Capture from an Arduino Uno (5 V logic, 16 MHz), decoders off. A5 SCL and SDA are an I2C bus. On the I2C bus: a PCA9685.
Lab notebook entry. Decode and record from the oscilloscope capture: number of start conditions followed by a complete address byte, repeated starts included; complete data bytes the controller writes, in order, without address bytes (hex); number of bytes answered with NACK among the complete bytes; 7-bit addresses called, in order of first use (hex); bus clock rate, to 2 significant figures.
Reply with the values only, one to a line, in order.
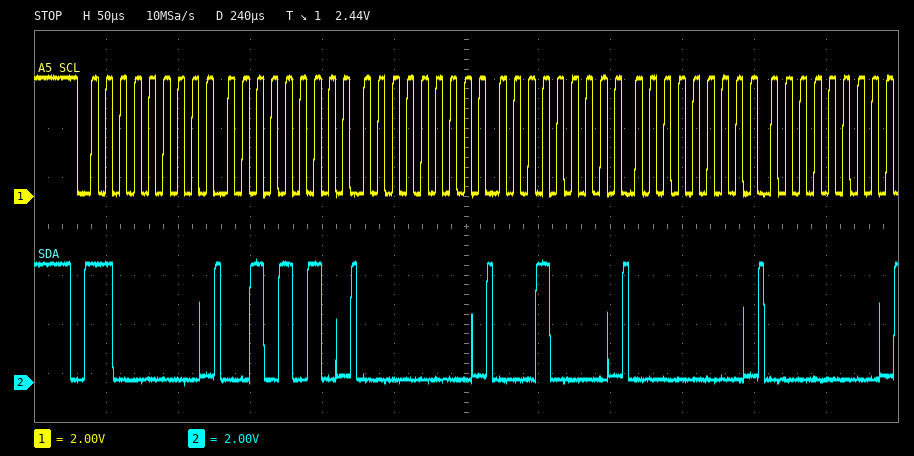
1
2A 00 10 00 00
0
0x60
100 kHz
